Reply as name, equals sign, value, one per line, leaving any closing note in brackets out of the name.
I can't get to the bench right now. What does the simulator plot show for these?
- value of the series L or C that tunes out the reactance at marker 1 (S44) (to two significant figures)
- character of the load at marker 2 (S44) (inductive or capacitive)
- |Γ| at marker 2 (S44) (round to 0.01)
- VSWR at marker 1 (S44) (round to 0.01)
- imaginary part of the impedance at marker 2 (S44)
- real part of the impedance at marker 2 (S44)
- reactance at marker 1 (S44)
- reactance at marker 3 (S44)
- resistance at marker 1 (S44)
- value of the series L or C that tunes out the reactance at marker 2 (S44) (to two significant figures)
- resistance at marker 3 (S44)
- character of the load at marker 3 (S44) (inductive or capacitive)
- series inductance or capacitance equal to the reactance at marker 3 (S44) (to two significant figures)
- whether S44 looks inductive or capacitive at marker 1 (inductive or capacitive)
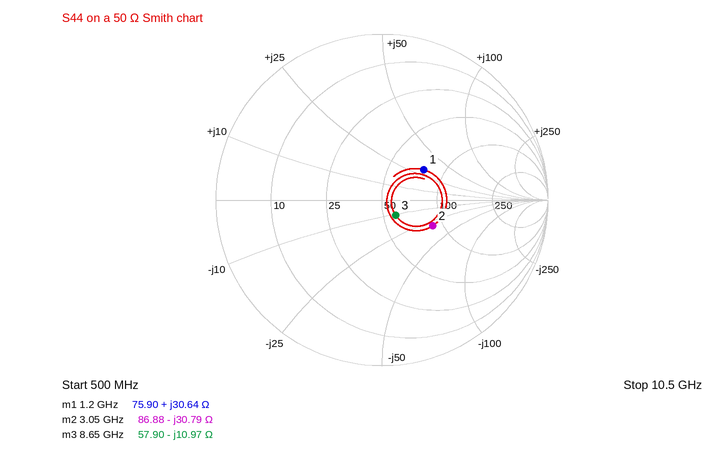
value of the series L or C that tunes out the reactance at marker 1 (S44) = 4.3 pF
character of the load at marker 2 (S44) = capacitive
|Γ| at marker 2 (S44) = 0.34
VSWR at marker 1 (S44) = 1.90
imaginary part of the impedance at marker 2 = -30.79 Ω
real part of the impedance at marker 2 = 86.88 Ω
reactance at marker 1 = +30.64 Ω
reactance at marker 3 = -10.97 Ω
resistance at marker 1 = 75.90 Ω
value of the series L or C that tunes out the reactance at marker 2 (S44) = 1.6 nH
resistance at marker 3 = 57.90 Ω
character of the load at marker 3 (S44) = capacitive
series inductance or capacitance equal to the reactance at marker 3 (S44) = 1.7 pF
whether S44 looks inductive or capacitive at marker 1 = inductive
